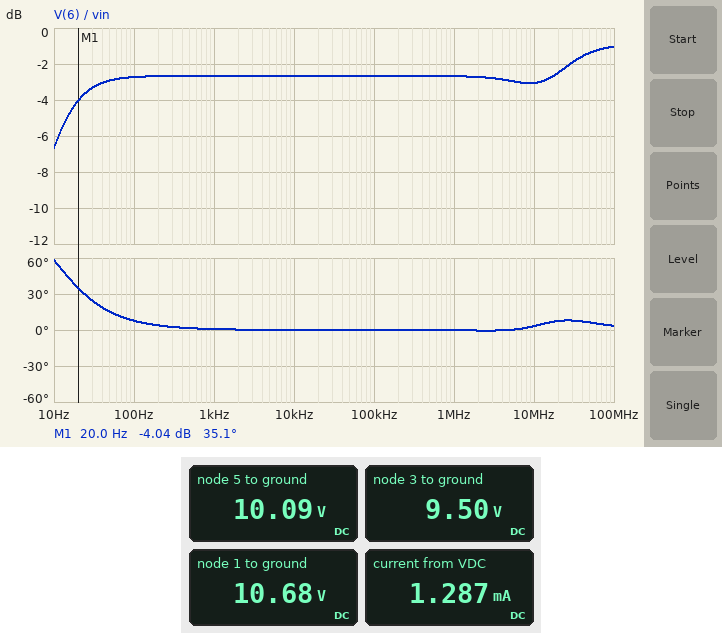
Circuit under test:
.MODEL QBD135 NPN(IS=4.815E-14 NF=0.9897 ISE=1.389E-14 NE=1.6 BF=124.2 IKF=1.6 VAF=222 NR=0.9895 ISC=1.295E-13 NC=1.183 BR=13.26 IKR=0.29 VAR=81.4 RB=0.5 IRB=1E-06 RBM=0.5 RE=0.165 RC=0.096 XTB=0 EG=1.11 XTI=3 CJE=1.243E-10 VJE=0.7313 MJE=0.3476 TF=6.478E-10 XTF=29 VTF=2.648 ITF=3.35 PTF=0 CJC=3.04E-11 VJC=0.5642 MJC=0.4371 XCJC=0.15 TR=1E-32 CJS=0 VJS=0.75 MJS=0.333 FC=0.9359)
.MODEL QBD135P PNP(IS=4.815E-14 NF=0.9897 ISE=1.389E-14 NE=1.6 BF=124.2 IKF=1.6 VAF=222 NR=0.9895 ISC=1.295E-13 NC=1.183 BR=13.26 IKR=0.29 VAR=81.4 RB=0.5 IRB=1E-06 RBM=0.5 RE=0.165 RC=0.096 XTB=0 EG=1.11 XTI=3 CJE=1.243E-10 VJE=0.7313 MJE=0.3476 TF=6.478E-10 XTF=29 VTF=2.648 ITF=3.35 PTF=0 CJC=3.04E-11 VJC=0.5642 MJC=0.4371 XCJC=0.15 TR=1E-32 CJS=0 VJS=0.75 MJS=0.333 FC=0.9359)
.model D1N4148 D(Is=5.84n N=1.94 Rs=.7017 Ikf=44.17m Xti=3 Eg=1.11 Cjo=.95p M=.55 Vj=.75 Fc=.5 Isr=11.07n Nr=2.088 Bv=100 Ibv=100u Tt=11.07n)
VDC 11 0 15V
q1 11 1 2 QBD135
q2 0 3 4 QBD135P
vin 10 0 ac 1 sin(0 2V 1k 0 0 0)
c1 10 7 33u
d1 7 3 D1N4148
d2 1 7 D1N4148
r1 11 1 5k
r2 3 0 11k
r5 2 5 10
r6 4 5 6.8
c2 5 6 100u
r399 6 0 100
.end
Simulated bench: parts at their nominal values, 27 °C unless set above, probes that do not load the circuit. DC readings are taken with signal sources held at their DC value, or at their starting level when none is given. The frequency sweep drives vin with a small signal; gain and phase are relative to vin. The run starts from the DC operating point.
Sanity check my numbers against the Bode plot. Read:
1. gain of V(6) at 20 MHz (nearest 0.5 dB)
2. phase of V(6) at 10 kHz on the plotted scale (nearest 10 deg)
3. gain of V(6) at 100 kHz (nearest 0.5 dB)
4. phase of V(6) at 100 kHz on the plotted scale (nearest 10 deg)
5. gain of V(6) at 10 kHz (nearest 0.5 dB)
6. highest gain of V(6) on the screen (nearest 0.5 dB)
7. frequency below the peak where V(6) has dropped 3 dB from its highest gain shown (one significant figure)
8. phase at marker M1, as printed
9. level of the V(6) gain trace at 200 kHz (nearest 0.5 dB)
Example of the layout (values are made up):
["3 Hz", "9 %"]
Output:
["-2.5 dB", "0 deg", "-2.5 dB", "0 deg", "-2.5 dB", "-1.0 dB", "20 Hz", "35.1 deg", "-2.5 dB"]
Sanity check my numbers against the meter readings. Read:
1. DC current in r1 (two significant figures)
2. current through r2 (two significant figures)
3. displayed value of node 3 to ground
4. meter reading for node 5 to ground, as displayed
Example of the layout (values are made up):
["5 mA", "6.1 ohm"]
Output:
["860 µA", "860 µA", "9.50 V", "10.09 V"]
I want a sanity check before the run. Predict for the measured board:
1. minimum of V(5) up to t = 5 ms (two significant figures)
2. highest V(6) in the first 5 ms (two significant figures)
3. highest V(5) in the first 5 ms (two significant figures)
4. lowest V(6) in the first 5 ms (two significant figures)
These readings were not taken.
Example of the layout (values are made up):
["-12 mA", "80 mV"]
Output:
["8.3 V", "1.7 V", "12 V", "-1.8 V"]
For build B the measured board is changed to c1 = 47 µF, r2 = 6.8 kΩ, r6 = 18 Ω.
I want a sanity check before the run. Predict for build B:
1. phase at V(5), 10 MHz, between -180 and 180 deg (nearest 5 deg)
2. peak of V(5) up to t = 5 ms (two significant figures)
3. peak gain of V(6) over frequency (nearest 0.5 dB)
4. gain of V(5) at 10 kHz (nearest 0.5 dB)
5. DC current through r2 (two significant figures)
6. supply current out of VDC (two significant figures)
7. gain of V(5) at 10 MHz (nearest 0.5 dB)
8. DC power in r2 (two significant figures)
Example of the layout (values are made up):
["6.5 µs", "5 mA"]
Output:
["0 deg", "10 V", "-1.0 dB", "-2.0 dB", "1.2 mA", "1.8 mA", "-2.5 dB", "9.3 mW"]
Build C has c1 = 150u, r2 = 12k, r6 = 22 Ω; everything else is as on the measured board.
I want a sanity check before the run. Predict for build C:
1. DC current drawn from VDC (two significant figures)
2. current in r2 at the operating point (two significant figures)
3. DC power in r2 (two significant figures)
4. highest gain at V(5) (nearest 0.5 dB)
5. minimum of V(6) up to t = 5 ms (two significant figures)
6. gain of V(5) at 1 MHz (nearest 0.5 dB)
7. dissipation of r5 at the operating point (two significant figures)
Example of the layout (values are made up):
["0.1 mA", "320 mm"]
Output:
["1.2 mA", "810 µA", "7.9 mW", "-0.5 dB", "-1.6 V", "-3.5 dB", "1.2 µW"]
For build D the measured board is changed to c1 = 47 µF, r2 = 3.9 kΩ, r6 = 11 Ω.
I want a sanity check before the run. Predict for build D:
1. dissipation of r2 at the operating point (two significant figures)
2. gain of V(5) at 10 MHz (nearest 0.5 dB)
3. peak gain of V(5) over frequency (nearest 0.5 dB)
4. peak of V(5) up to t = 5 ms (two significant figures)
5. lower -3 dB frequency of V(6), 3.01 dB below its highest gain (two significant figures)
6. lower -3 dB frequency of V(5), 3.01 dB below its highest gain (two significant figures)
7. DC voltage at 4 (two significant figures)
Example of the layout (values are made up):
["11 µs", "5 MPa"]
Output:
["9.3 mW", "-1.5 dB", "-0.5 dB", "8.4 V", "16 Hz", "1.4 Hz", "6.6 V"]
